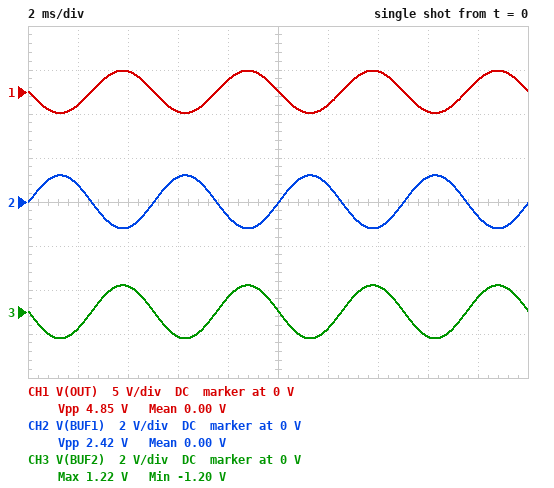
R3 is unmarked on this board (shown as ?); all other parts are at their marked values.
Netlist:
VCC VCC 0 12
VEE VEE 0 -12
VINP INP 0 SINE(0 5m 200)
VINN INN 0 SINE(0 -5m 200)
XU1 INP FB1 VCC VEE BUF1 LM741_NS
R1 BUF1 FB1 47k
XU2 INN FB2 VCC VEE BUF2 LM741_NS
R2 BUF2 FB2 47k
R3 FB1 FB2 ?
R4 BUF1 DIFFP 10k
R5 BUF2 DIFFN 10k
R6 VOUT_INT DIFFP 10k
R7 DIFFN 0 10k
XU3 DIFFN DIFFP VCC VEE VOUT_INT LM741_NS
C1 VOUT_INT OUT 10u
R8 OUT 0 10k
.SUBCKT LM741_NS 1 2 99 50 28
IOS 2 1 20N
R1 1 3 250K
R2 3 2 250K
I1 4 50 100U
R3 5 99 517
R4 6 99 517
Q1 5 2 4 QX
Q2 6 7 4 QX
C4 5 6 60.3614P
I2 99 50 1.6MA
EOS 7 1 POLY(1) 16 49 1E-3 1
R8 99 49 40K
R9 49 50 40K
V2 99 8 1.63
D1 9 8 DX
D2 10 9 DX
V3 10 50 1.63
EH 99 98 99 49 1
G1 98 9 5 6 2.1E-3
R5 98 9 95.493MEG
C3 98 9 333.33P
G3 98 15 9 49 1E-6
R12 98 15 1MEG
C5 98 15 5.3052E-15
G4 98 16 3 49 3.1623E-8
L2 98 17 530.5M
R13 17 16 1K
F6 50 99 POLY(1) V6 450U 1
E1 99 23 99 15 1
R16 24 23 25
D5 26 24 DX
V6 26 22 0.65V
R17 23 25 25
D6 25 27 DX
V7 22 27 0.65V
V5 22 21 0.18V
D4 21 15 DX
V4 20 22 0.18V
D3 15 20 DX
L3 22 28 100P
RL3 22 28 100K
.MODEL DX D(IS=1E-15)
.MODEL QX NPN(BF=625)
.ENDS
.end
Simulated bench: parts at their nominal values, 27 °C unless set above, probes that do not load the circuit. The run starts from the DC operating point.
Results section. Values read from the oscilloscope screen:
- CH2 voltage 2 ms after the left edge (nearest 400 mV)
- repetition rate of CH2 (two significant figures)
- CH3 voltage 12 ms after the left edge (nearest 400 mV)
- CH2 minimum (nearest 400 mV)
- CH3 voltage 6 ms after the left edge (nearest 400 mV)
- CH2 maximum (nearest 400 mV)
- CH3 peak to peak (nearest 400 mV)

800 mV
200 Hz
-800 mV
-1.2 V
-1.2 V
1.2 V
2.4 V
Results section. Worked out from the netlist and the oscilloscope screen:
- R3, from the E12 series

390 Ω
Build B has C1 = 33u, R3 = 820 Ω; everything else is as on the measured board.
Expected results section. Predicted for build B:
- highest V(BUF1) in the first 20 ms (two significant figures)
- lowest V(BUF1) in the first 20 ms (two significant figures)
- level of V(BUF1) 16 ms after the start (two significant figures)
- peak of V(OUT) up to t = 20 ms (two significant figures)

580 mV
-570 mV
550 mV
1.2 V
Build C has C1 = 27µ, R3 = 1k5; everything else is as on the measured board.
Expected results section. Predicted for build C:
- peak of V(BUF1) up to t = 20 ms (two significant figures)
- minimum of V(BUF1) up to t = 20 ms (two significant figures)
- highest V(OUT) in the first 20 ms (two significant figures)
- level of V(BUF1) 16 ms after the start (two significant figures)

320 mV
-310 mV
640 mV
310 mV
